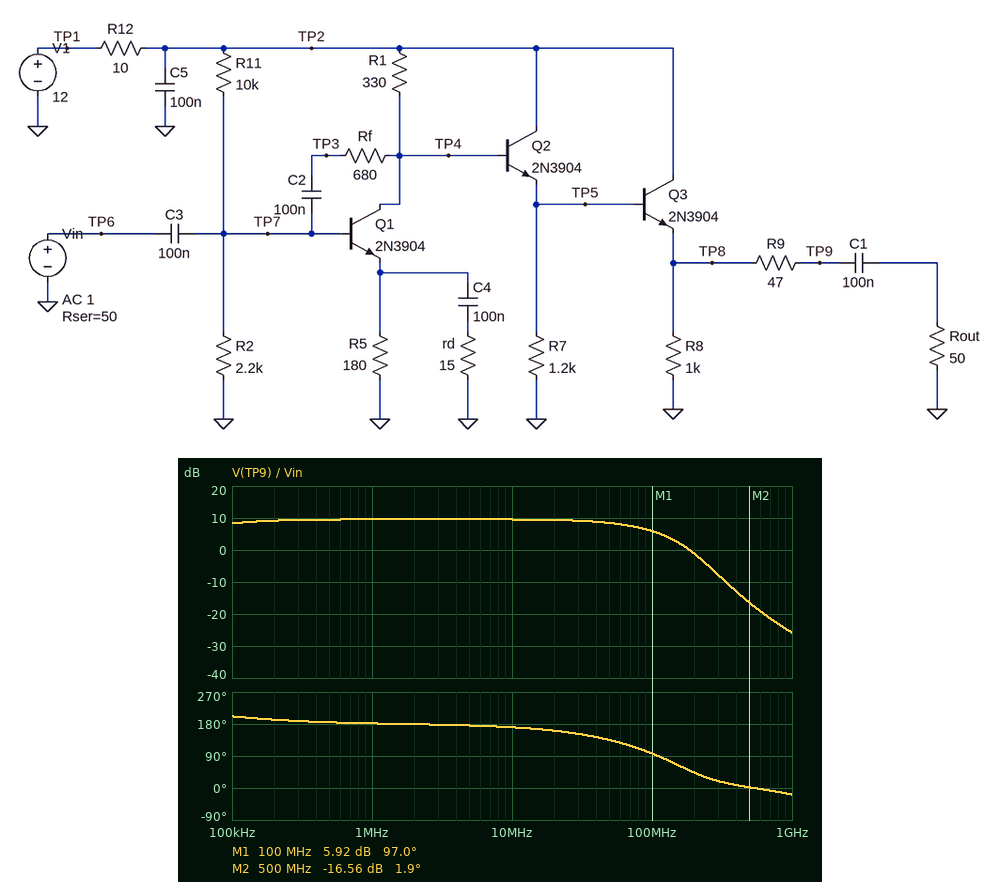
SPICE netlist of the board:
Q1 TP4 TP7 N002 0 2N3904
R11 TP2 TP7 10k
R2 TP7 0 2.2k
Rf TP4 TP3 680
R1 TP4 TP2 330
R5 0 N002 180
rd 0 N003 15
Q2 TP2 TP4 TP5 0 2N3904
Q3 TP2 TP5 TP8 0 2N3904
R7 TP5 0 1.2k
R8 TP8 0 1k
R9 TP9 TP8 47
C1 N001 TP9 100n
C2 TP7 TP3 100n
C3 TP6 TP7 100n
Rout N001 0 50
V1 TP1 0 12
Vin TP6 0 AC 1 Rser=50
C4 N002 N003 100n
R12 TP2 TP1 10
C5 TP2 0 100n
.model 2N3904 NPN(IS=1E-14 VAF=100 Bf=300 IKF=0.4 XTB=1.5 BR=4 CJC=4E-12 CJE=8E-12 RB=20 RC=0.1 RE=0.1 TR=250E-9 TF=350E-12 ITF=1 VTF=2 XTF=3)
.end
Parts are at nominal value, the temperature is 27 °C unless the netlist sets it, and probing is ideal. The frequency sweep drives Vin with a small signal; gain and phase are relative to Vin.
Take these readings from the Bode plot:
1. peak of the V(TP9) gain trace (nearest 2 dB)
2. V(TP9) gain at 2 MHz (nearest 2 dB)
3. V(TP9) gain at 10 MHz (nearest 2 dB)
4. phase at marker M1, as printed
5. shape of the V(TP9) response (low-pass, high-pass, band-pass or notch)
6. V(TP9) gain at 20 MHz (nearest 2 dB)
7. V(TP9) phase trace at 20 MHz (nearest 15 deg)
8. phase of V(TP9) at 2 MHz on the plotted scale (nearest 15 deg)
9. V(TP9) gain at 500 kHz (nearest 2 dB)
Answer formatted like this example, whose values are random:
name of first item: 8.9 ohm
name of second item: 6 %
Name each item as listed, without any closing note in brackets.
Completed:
peak of the V(TP9) gain trace: 10 dB
V(TP9) gain at 2 MHz: 10 dB
V(TP9) gain at 10 MHz: 10 dB
phase at marker M1, as printed: 97.0 deg
shape of the V(TP9) response: low-pass
V(TP9) gain at 20 MHz: 10 dB
V(TP9) phase trace at 20 MHz: 165 deg
phase of V(TP9) at 2 MHz on the plotted scale: 180 deg
V(TP9) gain at 500 kHz: 10 dB
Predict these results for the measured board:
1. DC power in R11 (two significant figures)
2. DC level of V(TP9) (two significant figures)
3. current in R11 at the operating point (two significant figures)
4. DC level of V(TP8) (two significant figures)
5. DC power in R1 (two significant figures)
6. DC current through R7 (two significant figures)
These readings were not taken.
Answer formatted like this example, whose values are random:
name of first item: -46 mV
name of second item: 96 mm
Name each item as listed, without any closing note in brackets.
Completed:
DC power in R11: 9.4 mW
DC level of V(TP9): 7.8 V
current in R11 at the operating point: 970 µA
DC level of V(TP8): 7.8 V
DC power in R1: 19 mW
DC current through R7: 7.1 mA
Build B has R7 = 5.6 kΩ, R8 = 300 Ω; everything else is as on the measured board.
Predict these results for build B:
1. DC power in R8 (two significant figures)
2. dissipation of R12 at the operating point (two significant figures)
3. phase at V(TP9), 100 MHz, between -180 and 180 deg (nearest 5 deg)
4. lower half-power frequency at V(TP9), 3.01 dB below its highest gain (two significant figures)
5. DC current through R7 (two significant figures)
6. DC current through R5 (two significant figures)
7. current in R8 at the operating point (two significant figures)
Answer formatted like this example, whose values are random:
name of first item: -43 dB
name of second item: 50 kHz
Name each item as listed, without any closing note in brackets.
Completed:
DC power in R8: 200 mW
dissipation of R12 at the operating point: 13 mW
phase at V(TP9), 100 MHz, between -180 and 180 deg: 90 deg
lower half-power frequency at V(TP9), 3.01 dB below its highest gain: 54 kHz
DC current through R7: 1.5 mA
DC current through R5: 7.5 mA
current in R8 at the operating point: 26 mA
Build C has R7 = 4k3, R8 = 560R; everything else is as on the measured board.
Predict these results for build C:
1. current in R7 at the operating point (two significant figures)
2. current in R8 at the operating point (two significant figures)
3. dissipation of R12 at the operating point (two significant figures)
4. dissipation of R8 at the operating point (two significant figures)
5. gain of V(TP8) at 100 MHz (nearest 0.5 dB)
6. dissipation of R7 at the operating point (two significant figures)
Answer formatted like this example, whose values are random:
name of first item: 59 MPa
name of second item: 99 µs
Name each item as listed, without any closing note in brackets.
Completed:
current in R7 at the operating point: 2.0 mA
current in R8 at the operating point: 14 mA
dissipation of R12 at the operating point: 6.0 mW
dissipation of R8 at the operating point: 110 mW
gain of V(TP8) at 100 MHz: 12.0 dB
dissipation of R7 at the operating point: 17 mW
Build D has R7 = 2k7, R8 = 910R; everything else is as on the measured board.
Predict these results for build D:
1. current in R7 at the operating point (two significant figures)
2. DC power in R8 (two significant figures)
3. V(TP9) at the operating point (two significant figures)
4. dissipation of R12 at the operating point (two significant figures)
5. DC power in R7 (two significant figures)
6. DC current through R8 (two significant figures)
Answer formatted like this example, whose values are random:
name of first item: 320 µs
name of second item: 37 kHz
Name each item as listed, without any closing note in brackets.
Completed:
current in R7 at the operating point: 3.2 mA
DC power in R8: 68 mW
V(TP9) at the operating point: 7.9 V
dissipation of R12 at the operating point: 4.2 mW
DC power in R7: 27 mW
DC current through R8: 8.7 mA
